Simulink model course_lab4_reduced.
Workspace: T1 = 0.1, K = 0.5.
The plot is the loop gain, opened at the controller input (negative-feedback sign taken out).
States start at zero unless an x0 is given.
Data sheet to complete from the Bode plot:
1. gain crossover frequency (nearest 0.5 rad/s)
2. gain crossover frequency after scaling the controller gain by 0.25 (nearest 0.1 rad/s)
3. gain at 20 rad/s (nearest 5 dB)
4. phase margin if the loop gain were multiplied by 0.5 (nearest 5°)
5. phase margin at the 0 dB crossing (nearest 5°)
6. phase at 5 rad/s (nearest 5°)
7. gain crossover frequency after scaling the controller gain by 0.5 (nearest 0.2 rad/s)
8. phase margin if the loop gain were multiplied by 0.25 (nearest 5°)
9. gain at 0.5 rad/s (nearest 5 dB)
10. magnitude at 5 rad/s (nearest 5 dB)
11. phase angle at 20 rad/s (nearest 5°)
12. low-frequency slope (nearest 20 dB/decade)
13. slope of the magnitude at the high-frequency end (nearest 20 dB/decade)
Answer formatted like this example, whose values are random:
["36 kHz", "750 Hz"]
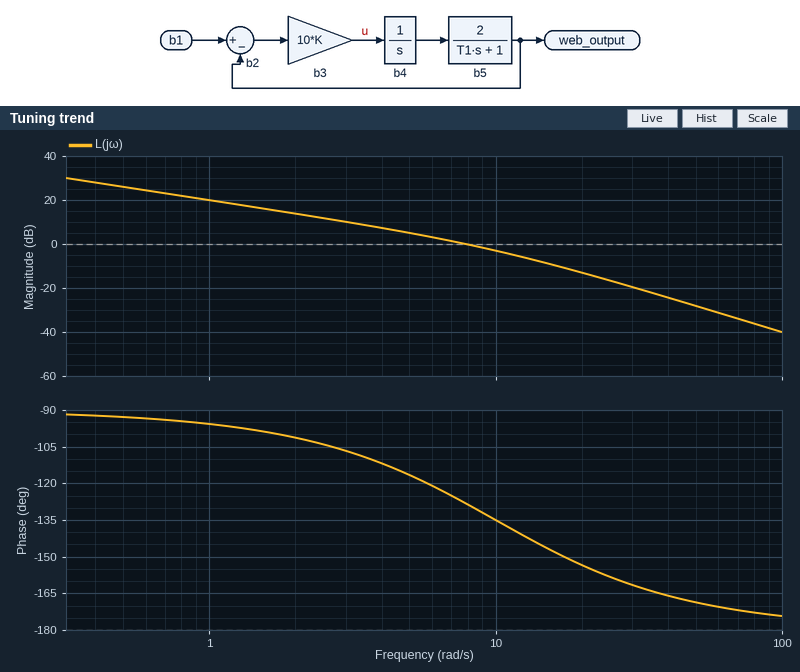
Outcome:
["8.0 rad/s", "2.4 rad/s", "-15 dB", "65°", "50°", "-115°", "4.6 rad/s", "75°", "25 dB", "5 dB", "-155°", "-20 dB/decade", "-40 dB/decade"]
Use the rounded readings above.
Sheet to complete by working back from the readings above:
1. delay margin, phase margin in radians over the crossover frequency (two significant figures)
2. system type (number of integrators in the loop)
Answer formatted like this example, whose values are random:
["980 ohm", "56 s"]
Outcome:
["0.11 s", "1"]
